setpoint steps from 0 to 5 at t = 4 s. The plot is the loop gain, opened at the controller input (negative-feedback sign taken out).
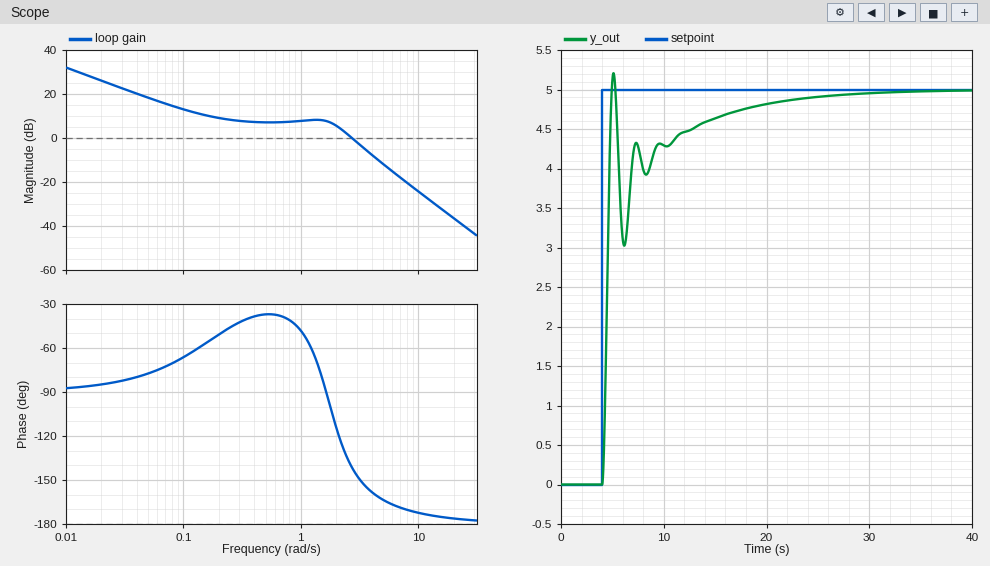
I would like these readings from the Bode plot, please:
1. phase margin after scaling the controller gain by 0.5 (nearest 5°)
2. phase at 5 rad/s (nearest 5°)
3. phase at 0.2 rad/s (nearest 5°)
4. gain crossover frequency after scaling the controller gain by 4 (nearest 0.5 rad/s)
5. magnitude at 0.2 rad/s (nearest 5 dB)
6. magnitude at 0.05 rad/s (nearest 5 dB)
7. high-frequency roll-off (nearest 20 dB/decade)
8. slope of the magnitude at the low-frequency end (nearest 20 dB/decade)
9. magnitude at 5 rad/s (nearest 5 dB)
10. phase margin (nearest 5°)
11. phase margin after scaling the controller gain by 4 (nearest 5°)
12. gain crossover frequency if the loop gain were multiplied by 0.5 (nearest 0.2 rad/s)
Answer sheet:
70°
-165°
-50°
5.0 rad/s
10 dB
20 dB
-40 dB/decade
-20 dB/decade
-10 dB
40°
15°
2.0 rad/s
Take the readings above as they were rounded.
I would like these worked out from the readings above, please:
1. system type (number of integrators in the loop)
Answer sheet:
1
